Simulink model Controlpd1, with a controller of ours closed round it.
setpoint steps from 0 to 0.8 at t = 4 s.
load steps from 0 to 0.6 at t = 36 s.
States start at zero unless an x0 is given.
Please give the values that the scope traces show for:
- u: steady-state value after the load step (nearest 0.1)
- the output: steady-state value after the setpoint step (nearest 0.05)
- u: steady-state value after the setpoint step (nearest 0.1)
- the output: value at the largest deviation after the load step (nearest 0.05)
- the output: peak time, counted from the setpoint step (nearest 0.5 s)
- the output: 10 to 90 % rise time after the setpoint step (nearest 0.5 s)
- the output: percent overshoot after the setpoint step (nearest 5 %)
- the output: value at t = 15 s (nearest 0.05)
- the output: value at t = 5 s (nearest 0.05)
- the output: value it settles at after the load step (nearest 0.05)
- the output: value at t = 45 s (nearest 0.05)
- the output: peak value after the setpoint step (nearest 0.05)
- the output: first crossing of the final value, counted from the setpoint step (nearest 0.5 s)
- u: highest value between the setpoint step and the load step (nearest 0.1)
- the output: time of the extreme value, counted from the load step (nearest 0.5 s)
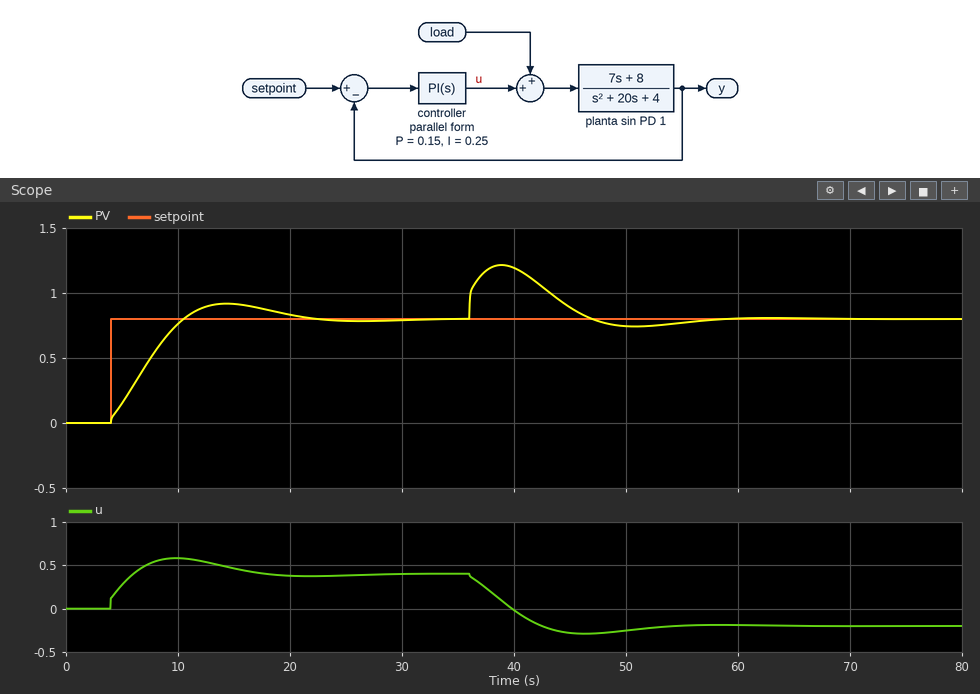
-0.2
0.80
0.4
1.20
10.5 s
5.0 s
15 %
0.90
0.15
0.80
0.90
0.90
6.5 s
0.6
3.0 s
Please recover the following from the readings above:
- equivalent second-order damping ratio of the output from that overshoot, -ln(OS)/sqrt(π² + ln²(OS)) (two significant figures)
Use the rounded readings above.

0.52
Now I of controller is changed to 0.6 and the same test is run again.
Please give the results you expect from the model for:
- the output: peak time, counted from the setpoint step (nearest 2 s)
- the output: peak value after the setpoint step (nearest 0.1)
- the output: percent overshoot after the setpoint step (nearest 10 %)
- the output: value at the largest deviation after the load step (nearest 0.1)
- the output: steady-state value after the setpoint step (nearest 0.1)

6 s
1.0
20 %
1.1
0.8
